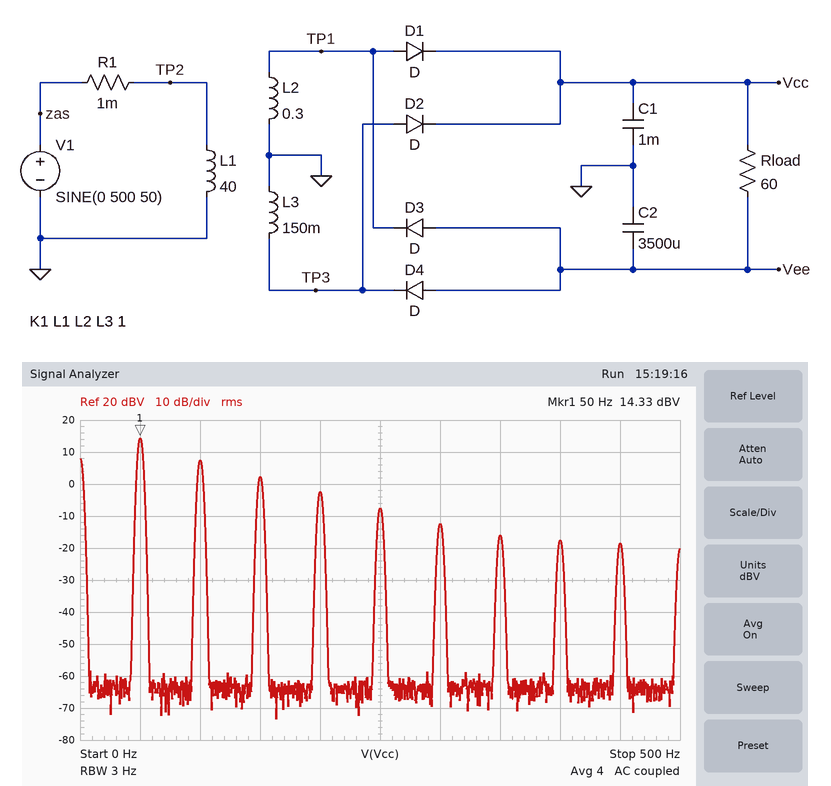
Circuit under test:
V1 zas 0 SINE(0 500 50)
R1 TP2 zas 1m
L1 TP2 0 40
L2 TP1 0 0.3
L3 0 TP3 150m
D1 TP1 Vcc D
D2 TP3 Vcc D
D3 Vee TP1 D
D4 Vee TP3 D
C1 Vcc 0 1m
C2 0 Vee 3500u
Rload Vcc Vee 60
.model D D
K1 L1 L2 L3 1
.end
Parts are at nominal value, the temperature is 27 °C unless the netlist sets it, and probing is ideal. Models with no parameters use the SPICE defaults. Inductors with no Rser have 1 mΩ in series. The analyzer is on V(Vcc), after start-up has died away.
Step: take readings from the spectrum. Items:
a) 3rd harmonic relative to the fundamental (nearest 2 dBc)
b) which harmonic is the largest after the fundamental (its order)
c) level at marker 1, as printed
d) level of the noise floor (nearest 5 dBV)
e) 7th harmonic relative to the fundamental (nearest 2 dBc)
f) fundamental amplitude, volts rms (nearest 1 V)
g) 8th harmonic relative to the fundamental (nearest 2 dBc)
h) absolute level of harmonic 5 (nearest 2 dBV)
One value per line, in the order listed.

-12 dBc
2
14.33 dBV
-65 dBV
-30 dBc
5 V
-32 dBc
-8 dBV
